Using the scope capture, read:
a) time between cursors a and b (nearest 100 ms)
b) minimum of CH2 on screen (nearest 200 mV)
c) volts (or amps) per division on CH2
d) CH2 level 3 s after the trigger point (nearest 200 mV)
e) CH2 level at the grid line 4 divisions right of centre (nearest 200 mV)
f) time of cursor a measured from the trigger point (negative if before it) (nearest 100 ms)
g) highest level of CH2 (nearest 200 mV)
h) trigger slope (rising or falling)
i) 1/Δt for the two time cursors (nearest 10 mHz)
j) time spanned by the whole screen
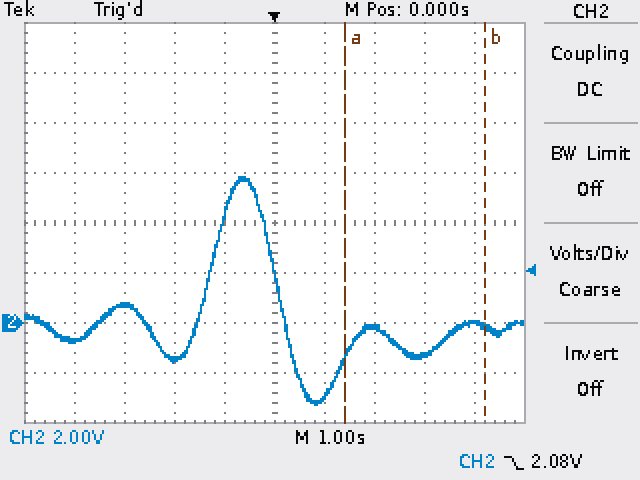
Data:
2.8 s
-3.2 V
2 V
-1.4 V
0.0 V
+1.4 s
5.8 V
falling
360 mHz
10 s
